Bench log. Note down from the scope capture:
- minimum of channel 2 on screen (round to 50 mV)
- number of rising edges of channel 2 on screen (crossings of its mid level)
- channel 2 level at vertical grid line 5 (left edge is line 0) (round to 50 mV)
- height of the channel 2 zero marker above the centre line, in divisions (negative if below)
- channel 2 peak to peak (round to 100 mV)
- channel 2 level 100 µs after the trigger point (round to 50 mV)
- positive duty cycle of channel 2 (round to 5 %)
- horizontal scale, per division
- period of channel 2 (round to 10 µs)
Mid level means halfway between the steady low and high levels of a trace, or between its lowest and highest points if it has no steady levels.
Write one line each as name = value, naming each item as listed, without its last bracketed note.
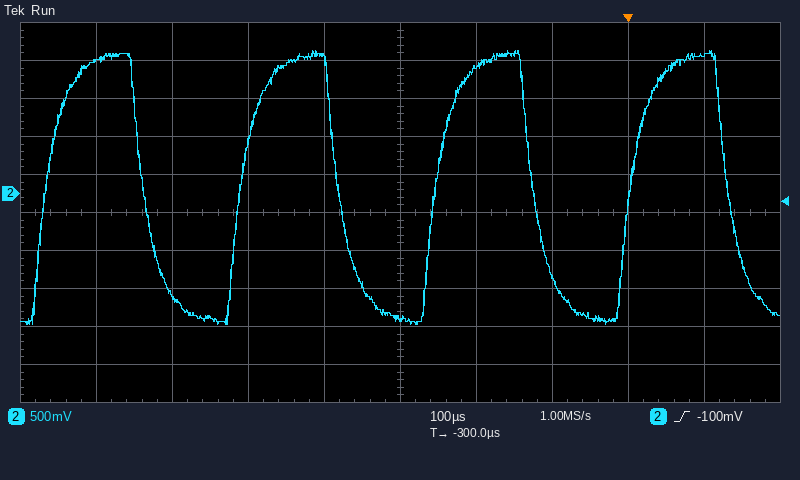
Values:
minimum of channel 2 on screen = -1.70 V
number of rising edges of channel 2 on screen = 4
channel 2 level at vertical grid line 5 (left edge is line 0) = -1.65 V
height of the channel 2 zero marker above the centre line, in divisions = +0.5 div
channel 2 peak to peak = 3.60 V
channel 2 level 100 µs after the trigger point = 1.80 V
positive duty cycle of channel 2 = 50 %
horizontal scale, per division = 100 µs
period of channel 2 = 260 µs
